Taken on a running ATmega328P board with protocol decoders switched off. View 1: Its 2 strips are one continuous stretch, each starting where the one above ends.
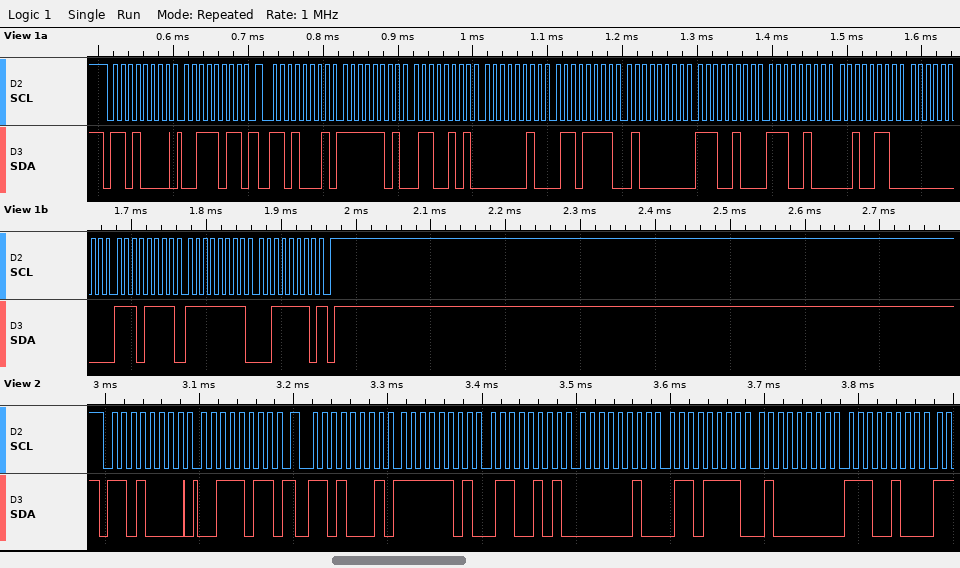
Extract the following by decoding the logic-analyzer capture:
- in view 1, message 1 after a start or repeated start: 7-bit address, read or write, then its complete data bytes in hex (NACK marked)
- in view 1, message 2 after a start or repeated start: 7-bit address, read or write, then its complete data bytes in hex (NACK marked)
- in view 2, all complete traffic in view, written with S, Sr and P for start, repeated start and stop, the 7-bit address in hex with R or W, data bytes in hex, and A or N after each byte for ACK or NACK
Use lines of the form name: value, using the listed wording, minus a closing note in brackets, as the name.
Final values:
in view 1, message 1 after a start or repeated start: 7-bit address, read or write, then its complete data bytes in hex: 0x68 write: 3B
in view 1, message 2 after a start or repeated start: 7-bit address, read or write, then its complete data bytes in hex: 0x68 read: FD 65 02 6F 40 E4 E4 26 00 EF FF 3E NACK
in view 2, all complete traffic in view, written with S, Sr and P for start, repeated start and stop, the 7-bit address in hex with R or W, data bytes in hex, and A or N after each byte for ACK or NACK: S 68W A 3B A Sr 68R A FD A 65 A 02 A 6F A 40 A E4 A
